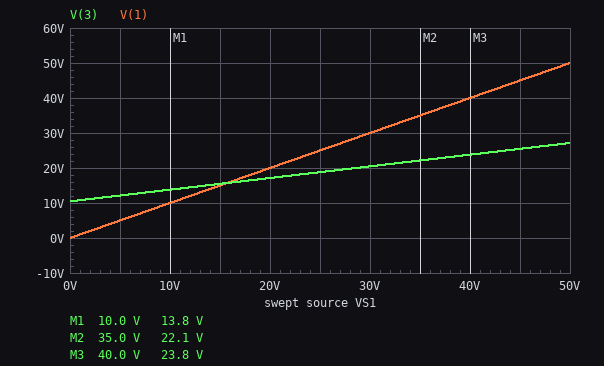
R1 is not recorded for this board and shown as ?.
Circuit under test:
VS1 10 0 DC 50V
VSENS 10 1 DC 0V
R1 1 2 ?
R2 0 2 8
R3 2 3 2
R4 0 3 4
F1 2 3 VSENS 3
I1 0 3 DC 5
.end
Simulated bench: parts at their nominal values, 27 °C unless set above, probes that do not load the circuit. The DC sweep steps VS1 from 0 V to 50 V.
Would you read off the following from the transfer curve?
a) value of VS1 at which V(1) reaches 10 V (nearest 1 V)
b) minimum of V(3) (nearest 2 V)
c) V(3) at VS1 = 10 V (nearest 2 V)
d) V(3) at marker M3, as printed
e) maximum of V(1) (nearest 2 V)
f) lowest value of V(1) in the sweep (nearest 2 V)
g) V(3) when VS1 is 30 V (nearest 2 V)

10 V
10 V
14 V
23.8 V
50 V
0 V
20 V
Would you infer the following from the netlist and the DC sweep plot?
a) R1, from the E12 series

12 Ω
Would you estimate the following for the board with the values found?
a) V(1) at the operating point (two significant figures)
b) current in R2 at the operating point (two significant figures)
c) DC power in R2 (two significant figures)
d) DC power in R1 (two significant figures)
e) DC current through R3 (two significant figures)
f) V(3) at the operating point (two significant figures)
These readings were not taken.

50 V
1.4 A
16 W
120 W
7.9 A
27 V
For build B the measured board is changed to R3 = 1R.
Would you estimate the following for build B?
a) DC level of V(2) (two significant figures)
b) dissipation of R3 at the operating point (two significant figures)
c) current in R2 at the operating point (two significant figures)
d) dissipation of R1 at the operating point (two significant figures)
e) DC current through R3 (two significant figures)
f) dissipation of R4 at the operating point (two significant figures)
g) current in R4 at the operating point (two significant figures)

16 V
59 W
2.0 A
97 W
7.7 A
140 W
5.9 A
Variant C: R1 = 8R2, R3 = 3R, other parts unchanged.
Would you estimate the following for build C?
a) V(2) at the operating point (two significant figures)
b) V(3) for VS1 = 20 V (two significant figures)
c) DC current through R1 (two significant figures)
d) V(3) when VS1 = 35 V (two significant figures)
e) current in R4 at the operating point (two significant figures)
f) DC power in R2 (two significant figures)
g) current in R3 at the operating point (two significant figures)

4.8 V
21 V
5.5 A
30 V
9.9 A
2.9 W
12 A
